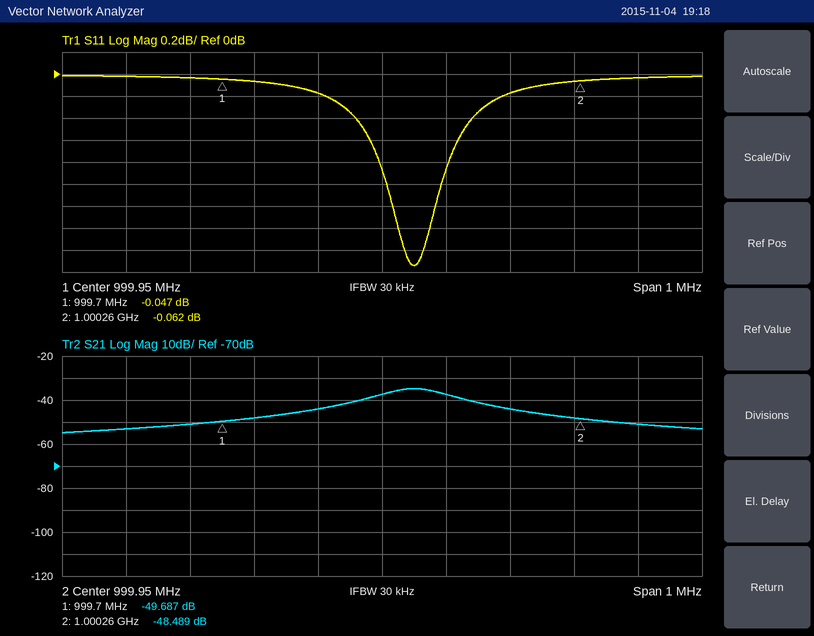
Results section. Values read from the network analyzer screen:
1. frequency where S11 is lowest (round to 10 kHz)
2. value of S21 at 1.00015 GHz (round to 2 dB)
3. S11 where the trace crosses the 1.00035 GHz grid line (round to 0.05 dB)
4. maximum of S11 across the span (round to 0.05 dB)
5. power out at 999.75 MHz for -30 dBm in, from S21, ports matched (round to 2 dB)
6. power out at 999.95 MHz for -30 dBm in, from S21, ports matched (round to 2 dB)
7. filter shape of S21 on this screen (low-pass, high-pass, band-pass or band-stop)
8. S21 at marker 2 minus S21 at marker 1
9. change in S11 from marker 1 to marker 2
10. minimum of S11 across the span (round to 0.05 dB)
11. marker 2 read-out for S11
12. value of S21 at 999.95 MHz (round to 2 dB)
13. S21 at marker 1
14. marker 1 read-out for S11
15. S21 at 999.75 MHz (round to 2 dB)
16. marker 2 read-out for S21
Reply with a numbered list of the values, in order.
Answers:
1. 1.00000 GHz
2. -44 dB
3. -0.05 dB
4. 0.00 dB
5. -78 dBm
6. -68 dBm
7. band-pass
8. 1.198 dB
9. -0.015 dB
10. -1.75 dB
11. -0.062 dB
12. -38 dB
13. -49.687 dB
14. -0.047 dB
15. -48 dB
16. -48.489 dB
